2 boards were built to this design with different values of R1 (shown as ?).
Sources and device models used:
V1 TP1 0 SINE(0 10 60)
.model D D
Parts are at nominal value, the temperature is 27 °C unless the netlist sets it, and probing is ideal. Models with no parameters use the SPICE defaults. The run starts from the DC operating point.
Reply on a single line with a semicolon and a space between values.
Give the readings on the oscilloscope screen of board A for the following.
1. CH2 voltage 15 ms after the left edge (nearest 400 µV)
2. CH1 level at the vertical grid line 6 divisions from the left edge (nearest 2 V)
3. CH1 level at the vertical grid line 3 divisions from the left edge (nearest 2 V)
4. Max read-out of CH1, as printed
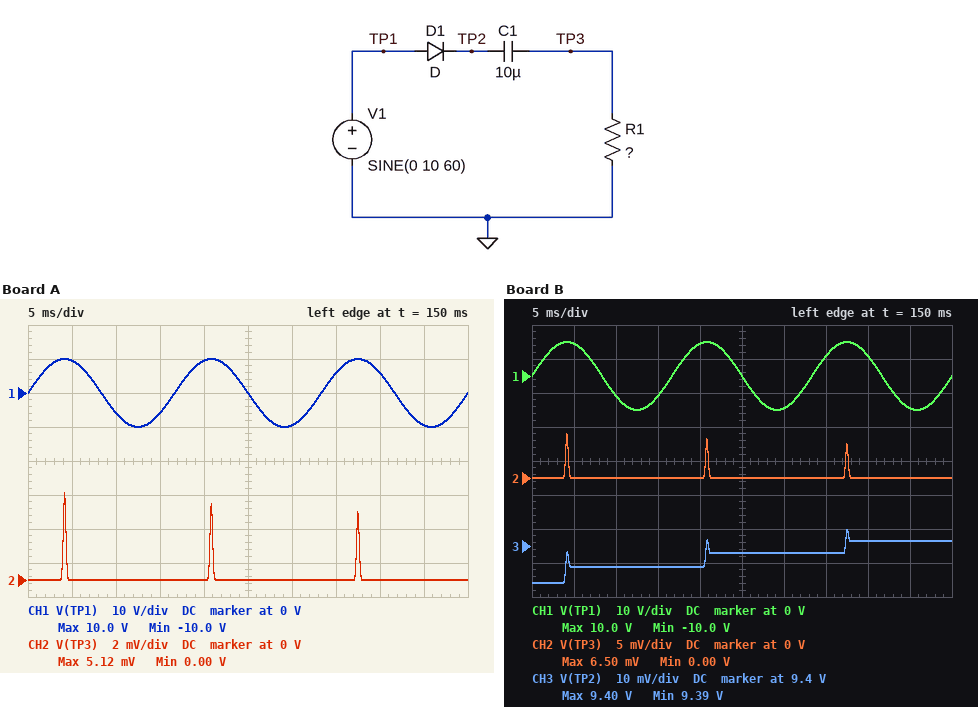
0 V; -10 V; -6 V; 10.0 V
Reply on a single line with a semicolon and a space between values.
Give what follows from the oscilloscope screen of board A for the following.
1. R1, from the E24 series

43 Ω
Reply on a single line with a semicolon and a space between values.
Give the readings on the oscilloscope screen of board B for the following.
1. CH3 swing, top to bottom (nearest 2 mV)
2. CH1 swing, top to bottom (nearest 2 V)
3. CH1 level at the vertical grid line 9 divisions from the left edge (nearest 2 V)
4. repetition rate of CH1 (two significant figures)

16 mV; 20 V; -10 V; 60 Hz
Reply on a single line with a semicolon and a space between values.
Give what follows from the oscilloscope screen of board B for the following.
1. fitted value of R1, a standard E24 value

51 Ω
